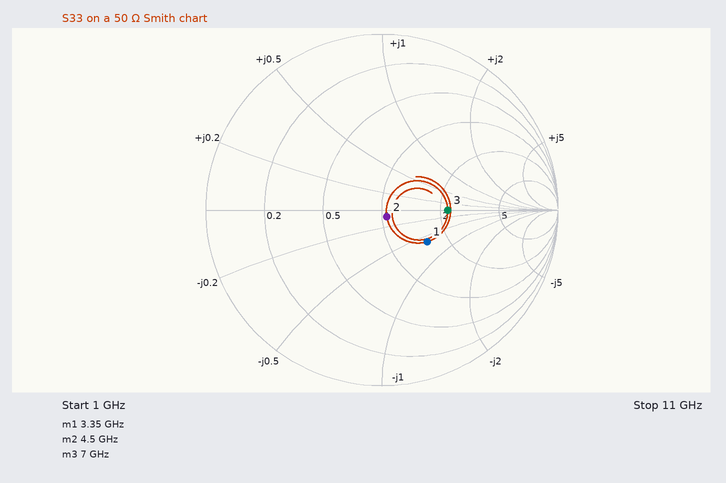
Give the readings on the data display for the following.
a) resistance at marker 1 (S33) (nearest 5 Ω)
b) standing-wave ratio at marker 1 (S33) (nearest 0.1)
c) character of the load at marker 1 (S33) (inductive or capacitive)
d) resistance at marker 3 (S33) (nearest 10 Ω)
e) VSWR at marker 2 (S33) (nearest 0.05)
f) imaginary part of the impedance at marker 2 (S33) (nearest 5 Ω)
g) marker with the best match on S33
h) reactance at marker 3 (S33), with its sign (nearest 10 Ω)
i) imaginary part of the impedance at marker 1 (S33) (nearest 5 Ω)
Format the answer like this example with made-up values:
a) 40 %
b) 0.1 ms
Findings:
a) 75 Ω
b) 1.9
c) capacitive
d) 110 Ω
e) 1.10
f) -5 Ω
g) marker 2
h) 0 Ω
i) -30 Ω
